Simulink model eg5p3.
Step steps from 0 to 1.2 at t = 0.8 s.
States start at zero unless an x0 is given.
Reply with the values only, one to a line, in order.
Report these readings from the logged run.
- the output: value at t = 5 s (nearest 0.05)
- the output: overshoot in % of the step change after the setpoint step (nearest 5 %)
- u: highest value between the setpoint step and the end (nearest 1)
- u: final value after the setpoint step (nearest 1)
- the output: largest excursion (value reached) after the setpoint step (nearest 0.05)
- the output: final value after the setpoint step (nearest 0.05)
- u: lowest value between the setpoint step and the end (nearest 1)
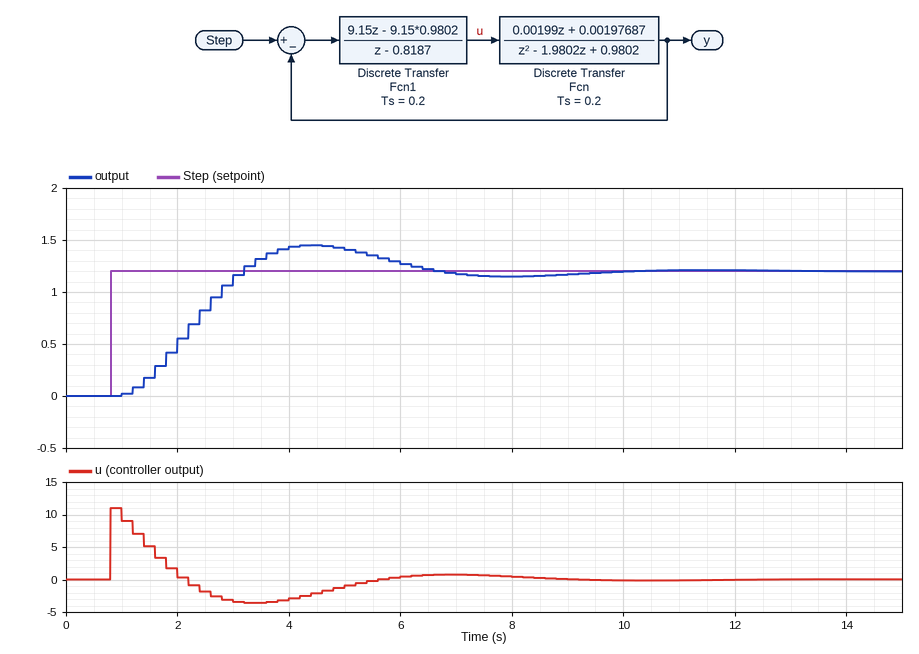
1.40
20 %
11
0
1.45
1.20
-4
